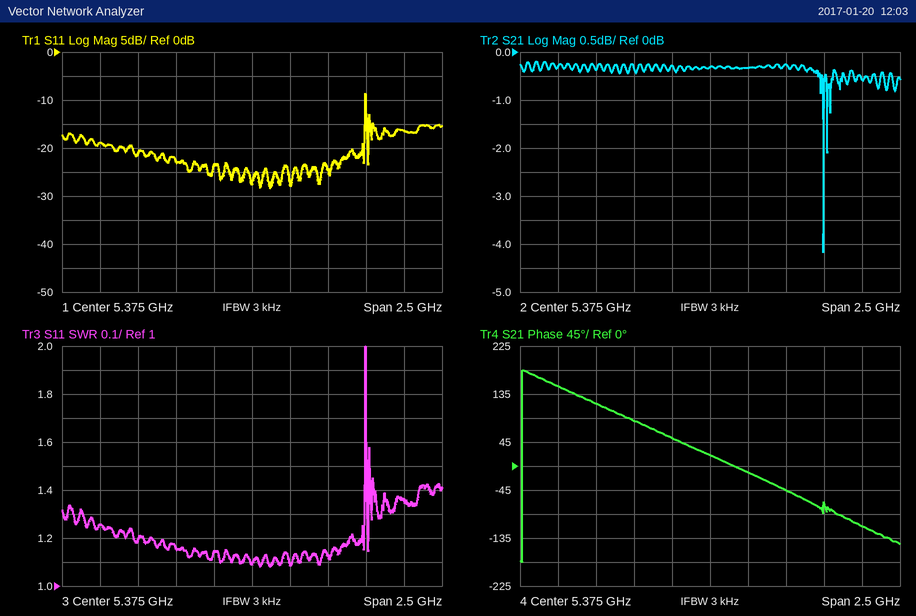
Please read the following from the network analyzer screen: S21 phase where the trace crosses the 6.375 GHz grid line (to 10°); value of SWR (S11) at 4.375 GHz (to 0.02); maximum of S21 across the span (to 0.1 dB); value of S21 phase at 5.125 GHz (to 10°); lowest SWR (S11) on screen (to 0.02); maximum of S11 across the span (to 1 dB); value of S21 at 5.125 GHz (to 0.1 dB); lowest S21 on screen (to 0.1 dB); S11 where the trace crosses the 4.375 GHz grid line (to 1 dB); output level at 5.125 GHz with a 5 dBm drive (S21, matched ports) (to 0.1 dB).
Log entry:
-110°
1.26
-0.2 dB
50°
1.08
-9 dB
-0.3 dB
-4.2 dB
-19 dB
4.7 dBm
